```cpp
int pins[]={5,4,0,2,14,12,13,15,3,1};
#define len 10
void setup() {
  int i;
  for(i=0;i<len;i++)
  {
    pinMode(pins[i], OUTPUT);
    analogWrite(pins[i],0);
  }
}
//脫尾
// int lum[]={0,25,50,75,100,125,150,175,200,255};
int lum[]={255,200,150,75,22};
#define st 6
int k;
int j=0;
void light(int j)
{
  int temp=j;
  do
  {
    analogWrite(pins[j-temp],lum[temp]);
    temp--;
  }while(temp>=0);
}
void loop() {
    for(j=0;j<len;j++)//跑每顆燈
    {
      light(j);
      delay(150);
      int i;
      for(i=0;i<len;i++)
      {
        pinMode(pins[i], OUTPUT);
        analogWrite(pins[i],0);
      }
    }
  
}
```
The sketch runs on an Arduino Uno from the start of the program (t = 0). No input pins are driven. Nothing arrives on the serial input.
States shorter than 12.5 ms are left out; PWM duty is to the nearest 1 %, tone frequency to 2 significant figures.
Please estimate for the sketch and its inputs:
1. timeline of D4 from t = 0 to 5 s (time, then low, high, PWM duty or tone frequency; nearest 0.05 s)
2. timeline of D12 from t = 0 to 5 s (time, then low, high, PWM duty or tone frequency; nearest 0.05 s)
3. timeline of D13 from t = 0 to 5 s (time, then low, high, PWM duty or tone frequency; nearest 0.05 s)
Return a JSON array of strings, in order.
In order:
["0 s low; 0.15 s high; 0.6 s low; 1.65 s high; 2.1 s low; 3.15 s high; 3.6 s low; 4.65 s high", "0 s low; 0.75 s high; 1.2 s low; 2.25 s high; 2.7 s low; 3.75 s high; 4.2 s low", "0 s low; 0.9 s high; 1.35 s low; 2.4 s high; 2.85 s low; 3.9 s high; 4.35 s low"]
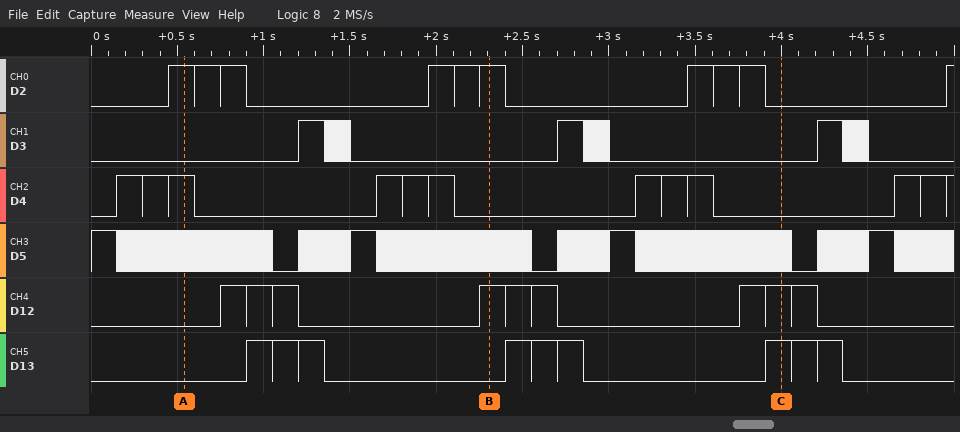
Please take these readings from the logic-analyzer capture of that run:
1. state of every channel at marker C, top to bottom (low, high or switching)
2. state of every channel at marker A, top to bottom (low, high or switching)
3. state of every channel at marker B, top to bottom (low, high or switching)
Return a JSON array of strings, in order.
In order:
["D2 low, D3 low, D4 low, D5 switching, D12 high, D13 high", "D2 high, D3 low, D4 high, D5 switching, D12 low, D13 low", "D2 high, D3 low, D4 low, D5 switching, D12 high, D13 low"]
